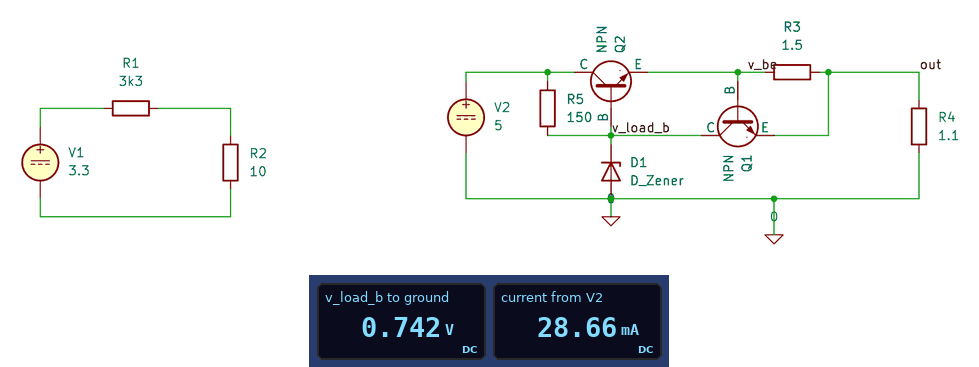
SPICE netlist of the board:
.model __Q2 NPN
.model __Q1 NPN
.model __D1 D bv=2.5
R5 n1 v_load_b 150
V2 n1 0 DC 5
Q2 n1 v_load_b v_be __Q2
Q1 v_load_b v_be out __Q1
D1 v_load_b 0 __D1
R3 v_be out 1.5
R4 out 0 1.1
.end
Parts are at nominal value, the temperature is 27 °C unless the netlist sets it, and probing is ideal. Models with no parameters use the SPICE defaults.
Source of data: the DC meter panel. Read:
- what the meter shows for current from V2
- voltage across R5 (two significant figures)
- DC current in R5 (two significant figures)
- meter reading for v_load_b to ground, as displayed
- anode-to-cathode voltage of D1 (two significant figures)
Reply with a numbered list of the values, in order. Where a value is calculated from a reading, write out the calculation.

1. 28.66 mA
2. 5 V - 742 mV = 4.3 V
3. (5 V - 742 mV) / 150 Ω = 28 mA
4. 0.742 V
5. 742 mV = 740 mV
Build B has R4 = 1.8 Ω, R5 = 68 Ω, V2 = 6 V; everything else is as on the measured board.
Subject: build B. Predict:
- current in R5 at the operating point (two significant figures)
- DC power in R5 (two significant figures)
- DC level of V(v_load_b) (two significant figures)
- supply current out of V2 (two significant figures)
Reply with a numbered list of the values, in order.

1. 77 mA
2. 400 mW
3. 770 mV
4. 78 mA
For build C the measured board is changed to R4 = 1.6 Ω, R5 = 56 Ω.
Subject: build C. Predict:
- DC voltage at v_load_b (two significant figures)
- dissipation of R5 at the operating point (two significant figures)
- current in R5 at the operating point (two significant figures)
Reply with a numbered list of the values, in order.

1. 770 mV
2. 320 mW
3. 76 mA
